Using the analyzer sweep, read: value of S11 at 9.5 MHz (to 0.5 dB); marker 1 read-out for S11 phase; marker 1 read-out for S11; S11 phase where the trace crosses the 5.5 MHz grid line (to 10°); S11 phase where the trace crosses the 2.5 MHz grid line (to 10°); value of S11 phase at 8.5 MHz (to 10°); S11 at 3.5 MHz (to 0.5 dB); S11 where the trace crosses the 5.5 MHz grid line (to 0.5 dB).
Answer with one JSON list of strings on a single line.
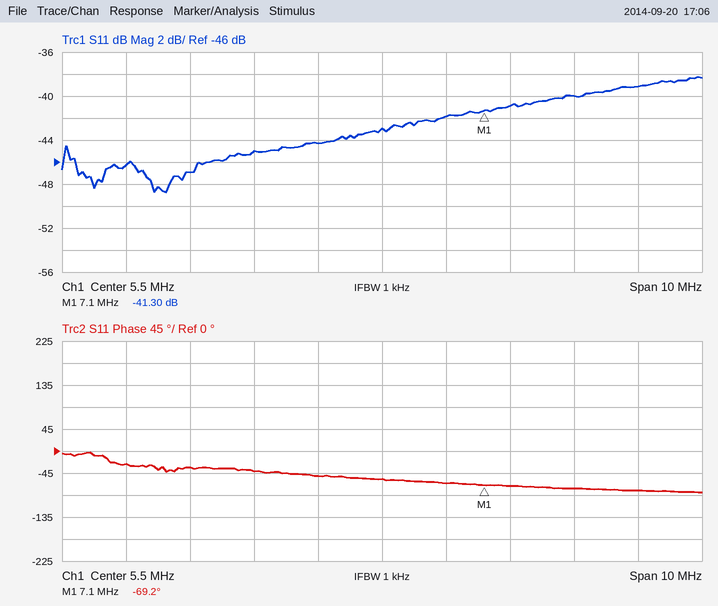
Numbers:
["-39.0 dB", "-69.2°", "-41.30 dB", "-60°", "-30°", "-80°", "-45.0 dB", "-43.0 dB"]
